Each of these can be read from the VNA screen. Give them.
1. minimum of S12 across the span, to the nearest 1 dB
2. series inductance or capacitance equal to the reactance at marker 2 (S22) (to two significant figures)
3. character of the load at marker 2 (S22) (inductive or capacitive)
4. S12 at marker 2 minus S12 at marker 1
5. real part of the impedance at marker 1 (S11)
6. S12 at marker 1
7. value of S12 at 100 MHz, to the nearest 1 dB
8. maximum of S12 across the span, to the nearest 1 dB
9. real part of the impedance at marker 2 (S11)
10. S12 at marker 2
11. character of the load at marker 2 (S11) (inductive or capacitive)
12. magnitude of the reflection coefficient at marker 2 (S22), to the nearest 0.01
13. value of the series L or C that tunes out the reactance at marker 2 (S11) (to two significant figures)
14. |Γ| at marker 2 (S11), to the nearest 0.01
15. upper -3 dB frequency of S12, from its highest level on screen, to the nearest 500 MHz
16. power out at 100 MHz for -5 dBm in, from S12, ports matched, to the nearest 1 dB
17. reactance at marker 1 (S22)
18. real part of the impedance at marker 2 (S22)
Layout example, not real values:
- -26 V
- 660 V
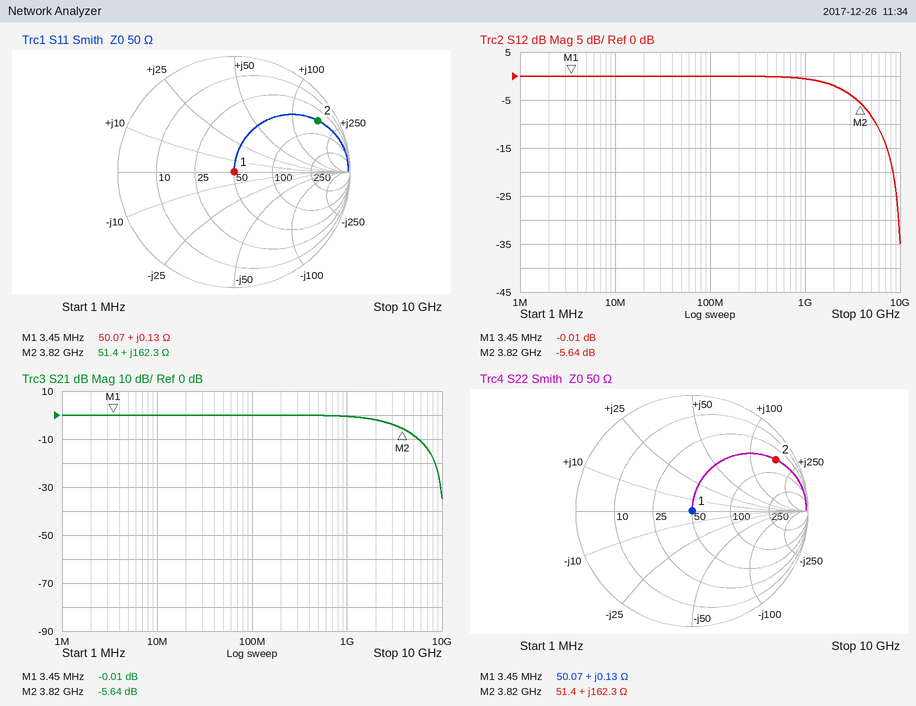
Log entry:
- -35 dB
- 6.8 nH
- inductive
- -5.63 dB
- 50.07 Ω
- -0.01 dB
- 0 dB
- 0 dB
- 51.4 Ω
- -5.64 dB
- inductive
- 0.85
- 260 fF
- 0.85
- 2.5 GHz
- -5 dBm
- +0.13 Ω
- 51.4 Ω
